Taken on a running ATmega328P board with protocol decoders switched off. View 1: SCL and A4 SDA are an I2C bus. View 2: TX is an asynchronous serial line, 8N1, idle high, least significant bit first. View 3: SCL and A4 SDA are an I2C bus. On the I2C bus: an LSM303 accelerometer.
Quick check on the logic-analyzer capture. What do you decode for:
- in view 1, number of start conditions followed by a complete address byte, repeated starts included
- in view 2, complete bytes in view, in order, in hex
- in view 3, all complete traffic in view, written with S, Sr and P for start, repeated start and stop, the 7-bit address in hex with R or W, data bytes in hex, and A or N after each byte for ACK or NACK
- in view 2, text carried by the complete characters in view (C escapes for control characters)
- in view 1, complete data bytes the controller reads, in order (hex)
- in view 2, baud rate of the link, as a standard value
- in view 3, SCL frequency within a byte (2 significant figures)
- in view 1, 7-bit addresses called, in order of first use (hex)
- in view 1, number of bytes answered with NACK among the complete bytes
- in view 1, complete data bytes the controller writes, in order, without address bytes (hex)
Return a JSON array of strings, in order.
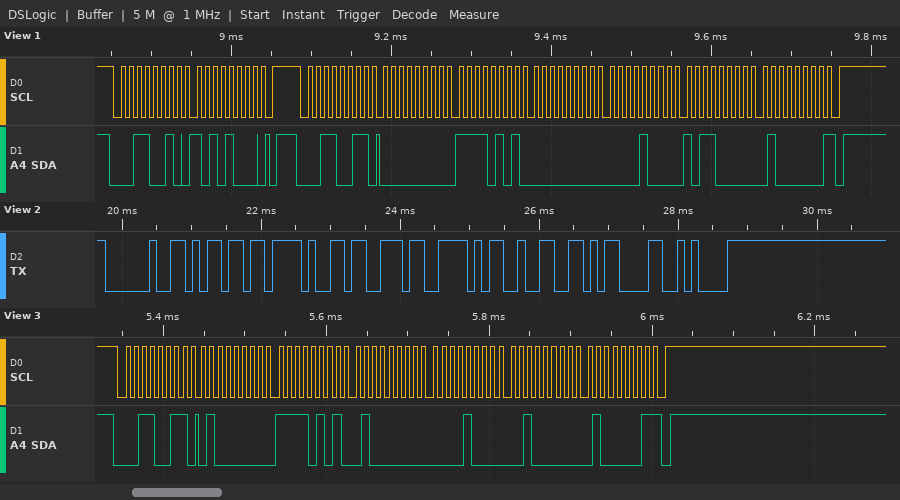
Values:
["2", "0x20 0x6D 0x2F 0x73 0x5E 0x32 0x0D 0x0A", "S 19R A 40 A F5 A 40 A 08 A 20 A 41 N P", "\" m/s^2\\r\\n\"", "00 F5 00 08 B0 40", "9600 baud", "100 kHz", "0x19", "1", "A8"]
